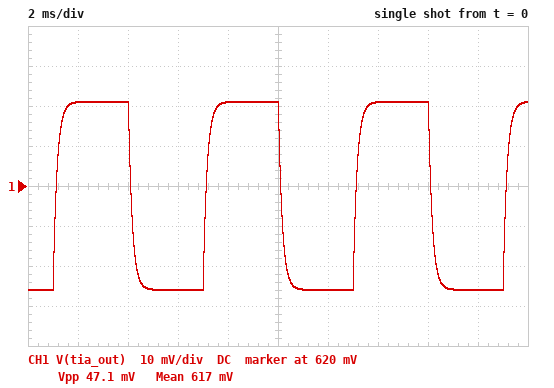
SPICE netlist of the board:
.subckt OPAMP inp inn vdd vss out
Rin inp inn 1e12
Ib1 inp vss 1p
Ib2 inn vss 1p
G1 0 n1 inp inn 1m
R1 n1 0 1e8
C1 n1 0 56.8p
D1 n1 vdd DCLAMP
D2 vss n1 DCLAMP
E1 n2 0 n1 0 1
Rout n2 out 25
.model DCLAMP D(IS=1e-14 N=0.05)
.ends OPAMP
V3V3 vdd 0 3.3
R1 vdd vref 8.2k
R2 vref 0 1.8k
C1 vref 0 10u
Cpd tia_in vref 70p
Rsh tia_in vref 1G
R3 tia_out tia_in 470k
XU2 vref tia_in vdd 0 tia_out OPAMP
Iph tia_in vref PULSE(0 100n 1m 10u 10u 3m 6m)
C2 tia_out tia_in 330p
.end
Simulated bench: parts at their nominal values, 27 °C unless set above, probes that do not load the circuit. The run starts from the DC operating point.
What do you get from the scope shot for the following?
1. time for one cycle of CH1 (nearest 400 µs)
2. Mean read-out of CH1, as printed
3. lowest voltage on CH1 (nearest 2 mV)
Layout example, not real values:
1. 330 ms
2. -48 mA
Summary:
1. 6.0 ms
2. 617 mV
3. 594 mV
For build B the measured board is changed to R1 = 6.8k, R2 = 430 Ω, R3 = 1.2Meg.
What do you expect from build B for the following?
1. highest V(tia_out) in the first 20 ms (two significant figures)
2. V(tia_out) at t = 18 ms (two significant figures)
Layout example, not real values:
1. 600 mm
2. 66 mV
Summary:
1. 320 mV
2. 200 mV
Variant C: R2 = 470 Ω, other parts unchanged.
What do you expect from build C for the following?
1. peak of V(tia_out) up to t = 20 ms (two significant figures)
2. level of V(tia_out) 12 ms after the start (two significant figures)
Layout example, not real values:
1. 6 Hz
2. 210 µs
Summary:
1. 230 mV
2. 180 mV
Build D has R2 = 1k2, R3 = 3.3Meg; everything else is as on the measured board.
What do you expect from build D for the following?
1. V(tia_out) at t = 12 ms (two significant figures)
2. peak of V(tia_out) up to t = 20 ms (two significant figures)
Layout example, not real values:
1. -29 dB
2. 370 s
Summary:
1. 470 mV
2. 730 mV
